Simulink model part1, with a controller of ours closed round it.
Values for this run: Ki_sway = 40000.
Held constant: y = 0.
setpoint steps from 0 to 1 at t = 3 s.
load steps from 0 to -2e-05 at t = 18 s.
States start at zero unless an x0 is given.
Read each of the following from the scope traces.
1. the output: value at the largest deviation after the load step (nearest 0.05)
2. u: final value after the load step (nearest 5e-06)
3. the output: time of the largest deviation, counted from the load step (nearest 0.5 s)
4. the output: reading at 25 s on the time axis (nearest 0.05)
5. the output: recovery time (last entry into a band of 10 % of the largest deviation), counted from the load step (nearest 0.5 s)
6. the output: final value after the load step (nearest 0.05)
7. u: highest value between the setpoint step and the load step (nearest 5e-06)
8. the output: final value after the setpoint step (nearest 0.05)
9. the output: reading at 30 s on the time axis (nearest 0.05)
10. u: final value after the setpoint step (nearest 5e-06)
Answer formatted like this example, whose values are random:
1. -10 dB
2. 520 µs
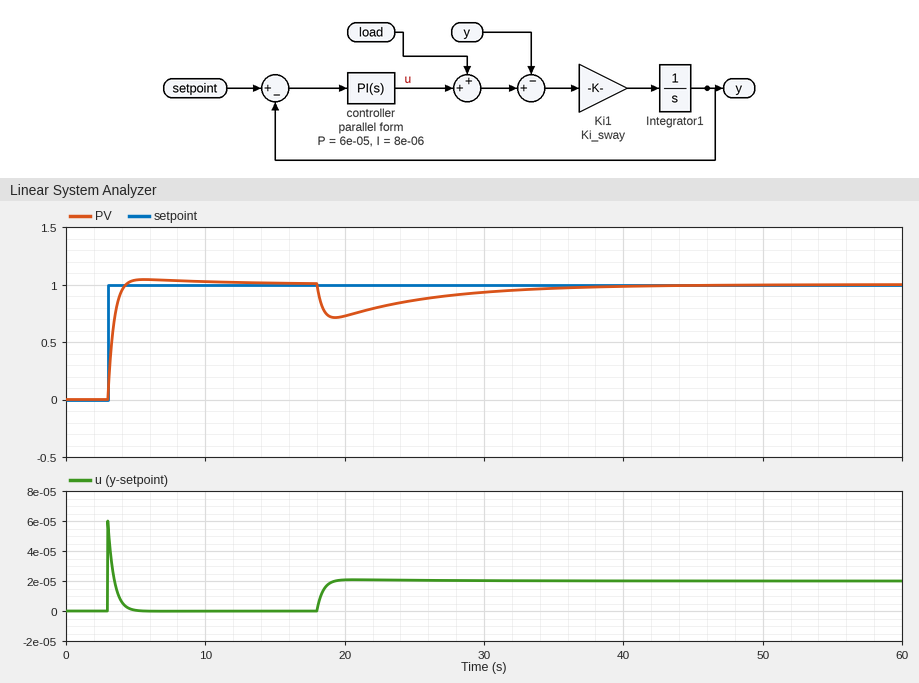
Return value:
1. 0.70
2. 0.000020
3. 1.5 s
4. 0.85
5. 18.0 s
6. 1.00
7. 0.000060
8. 1.00
9. 0.95
10. 0.000000
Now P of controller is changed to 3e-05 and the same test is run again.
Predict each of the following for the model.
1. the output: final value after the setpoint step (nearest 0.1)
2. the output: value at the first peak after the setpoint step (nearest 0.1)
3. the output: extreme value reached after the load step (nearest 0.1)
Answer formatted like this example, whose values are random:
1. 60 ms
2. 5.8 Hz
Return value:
1. 1.0
2. 1.1
3. 0.5
